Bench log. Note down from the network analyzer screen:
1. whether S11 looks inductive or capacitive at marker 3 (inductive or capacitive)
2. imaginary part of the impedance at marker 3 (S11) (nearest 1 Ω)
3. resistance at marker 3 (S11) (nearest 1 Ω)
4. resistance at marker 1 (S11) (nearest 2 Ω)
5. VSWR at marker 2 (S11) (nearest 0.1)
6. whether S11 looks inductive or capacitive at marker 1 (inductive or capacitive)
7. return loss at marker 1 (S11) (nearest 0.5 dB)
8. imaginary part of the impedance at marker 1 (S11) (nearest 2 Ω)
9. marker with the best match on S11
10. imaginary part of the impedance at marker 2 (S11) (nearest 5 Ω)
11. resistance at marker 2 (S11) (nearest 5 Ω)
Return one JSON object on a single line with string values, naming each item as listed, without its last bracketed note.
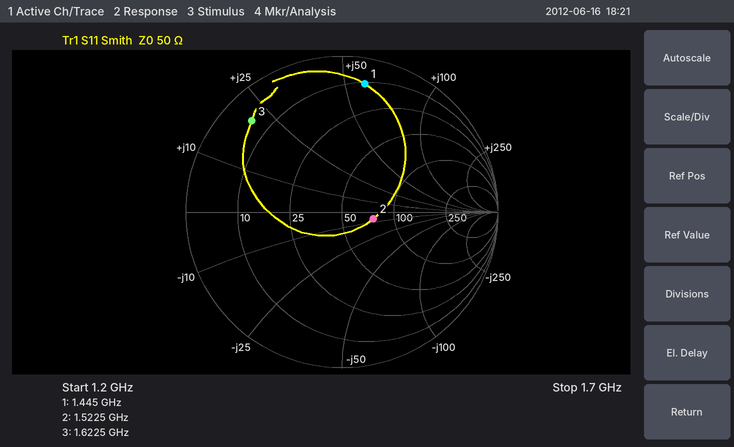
{"whether S11 looks inductive or capacitive at marker 3": "inductive", "imaginary part of the impedance at marker 3 (S11)": "+21 Ω", "resistance at marker 3 (S11)": "6 Ω", "resistance at marker 1 (S11)": "10 Ω", "VSWR at marker 2 (S11)": "1.5", "whether S11 looks inductive or capacitive at marker 1": "inductive", "return loss at marker 1 (S11)": "1.5 dB", "imaginary part of the impedance at marker 1 (S11)": "+58 Ω", "marker with the best match on S11": "marker 2", "imaginary part of the impedance at marker 2 (S11)": "-5 Ω", "resistance at marker 2 (S11)": "75 Ω"}
